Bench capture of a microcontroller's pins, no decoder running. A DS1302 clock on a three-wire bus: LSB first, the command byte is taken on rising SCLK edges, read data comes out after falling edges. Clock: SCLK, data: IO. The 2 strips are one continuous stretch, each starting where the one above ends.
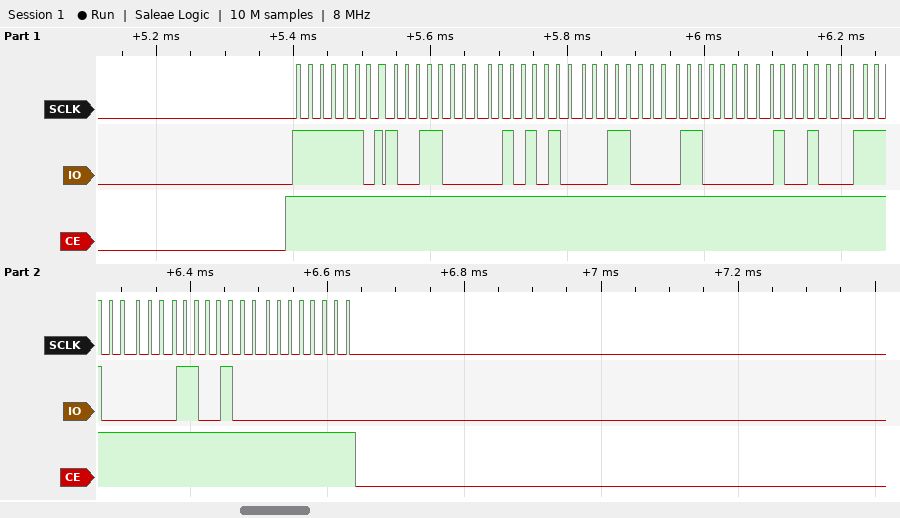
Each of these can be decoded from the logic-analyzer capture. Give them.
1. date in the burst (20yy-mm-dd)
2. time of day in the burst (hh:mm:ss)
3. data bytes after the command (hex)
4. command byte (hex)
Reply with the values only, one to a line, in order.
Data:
2026-12-06
18:54:19
19 54 18 06 12 07 26 00
0xBF
